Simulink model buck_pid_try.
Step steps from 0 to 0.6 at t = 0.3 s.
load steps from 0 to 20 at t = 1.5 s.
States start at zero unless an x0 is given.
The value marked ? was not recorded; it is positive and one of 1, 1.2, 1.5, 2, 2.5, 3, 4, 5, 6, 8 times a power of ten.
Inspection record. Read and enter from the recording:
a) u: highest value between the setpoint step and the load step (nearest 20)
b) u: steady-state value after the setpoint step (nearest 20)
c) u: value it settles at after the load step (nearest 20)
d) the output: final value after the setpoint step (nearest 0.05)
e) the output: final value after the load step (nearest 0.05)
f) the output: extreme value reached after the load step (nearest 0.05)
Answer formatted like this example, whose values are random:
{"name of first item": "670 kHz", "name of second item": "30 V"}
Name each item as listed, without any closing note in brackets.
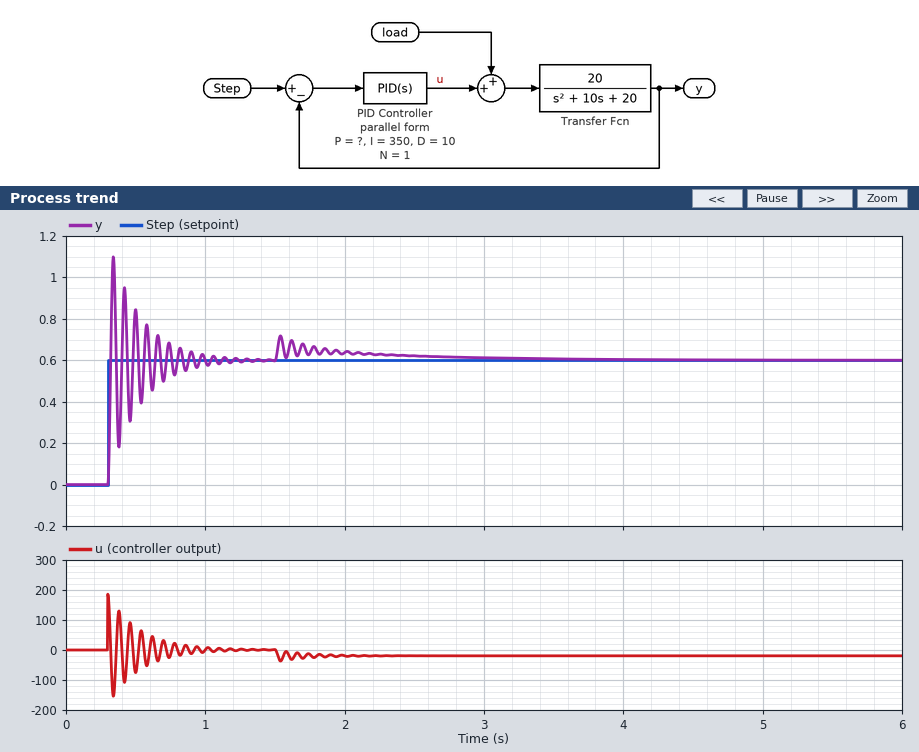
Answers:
{"u: highest value between the setpoint step and the load step": "180", "u: steady-state value after the setpoint step": "0", "u: value it settles at after the load step": "-20", "the output: final value after the setpoint step": "0.60", "the output: final value after the load step": "0.60", "the output: extreme value reached after the load step": "0.70"}
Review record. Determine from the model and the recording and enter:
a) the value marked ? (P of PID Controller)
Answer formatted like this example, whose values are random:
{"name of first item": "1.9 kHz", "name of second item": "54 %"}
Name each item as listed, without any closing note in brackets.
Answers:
{"the value marked ?": "300"}
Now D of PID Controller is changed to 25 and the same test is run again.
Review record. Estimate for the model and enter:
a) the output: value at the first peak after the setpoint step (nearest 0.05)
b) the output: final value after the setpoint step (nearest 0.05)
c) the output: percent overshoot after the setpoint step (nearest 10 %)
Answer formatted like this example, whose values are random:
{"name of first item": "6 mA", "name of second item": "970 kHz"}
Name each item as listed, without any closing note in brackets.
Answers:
{"the output: value at the first peak after the setpoint step": "1.10", "the output: final value after the setpoint step": "0.60", "the output: percent overshoot after the setpoint step": "80 %"}
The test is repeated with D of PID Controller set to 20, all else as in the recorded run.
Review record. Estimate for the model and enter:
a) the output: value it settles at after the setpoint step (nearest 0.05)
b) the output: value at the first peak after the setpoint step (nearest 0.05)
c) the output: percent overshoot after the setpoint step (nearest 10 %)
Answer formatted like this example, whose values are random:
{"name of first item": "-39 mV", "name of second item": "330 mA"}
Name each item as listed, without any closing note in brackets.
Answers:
{"the output: value it settles at after the setpoint step": "0.60", "the output: value at the first peak after the setpoint step": "1.10", "the output: percent overshoot after the setpoint step": "80 %"}
